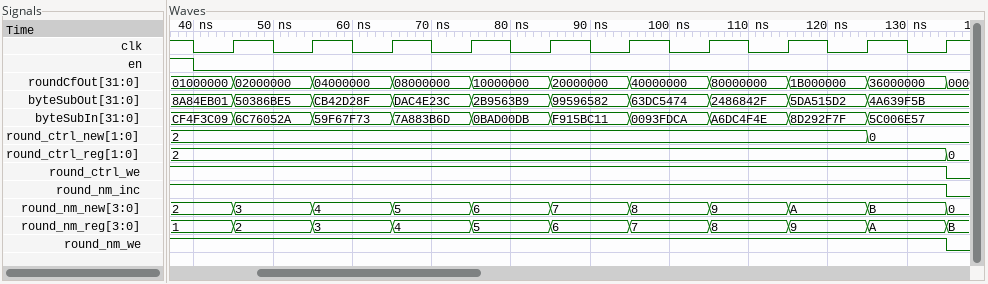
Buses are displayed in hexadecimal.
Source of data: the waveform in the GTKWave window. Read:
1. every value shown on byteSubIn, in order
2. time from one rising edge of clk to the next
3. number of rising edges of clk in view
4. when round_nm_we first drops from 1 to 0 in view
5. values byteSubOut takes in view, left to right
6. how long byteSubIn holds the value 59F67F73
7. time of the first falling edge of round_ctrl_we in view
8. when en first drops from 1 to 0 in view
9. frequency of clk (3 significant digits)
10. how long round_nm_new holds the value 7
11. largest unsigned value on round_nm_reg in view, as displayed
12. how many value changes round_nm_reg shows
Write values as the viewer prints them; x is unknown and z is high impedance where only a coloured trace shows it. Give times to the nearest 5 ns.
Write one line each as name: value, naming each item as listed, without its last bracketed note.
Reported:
every value shown on byteSubIn, in order: CF4F3C09, 6C76052A, 59F67F73, 7A883B6D, 0BAD00DB, F915BC11, 0093FDCA, A6DC4F4E, 8D292F7F, 5C006E57
time from one rising edge of clk to the next: 10 ns
number of rising edges of clk in view: 10
when round_nm_we first drops from 1 to 0 in view: 135 ns
values byteSubOut takes in view, left to right: 8A84EB01, 50386BE5, CB42D28F, DAC4E23C, 2B9563B9, 99596582, 63DC5474, 2486842F, 5DA515D2, 4A639F5B
how long byteSubIn holds the value 59F67F73: 10 ns
time of the first falling edge of round_ctrl_we in view: 135 ns
when en first drops from 1 to 0 in view: 40 ns
frequency of clk: 100 MHz
how long round_nm_new holds the value 7: 10 ns
largest unsigned value on round_nm_reg in view, as displayed: B
how many value changes round_nm_reg shows: 10
